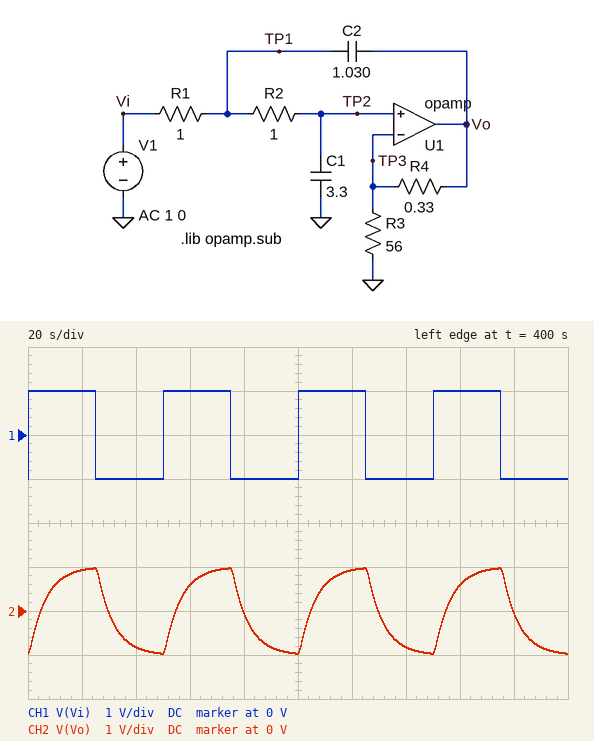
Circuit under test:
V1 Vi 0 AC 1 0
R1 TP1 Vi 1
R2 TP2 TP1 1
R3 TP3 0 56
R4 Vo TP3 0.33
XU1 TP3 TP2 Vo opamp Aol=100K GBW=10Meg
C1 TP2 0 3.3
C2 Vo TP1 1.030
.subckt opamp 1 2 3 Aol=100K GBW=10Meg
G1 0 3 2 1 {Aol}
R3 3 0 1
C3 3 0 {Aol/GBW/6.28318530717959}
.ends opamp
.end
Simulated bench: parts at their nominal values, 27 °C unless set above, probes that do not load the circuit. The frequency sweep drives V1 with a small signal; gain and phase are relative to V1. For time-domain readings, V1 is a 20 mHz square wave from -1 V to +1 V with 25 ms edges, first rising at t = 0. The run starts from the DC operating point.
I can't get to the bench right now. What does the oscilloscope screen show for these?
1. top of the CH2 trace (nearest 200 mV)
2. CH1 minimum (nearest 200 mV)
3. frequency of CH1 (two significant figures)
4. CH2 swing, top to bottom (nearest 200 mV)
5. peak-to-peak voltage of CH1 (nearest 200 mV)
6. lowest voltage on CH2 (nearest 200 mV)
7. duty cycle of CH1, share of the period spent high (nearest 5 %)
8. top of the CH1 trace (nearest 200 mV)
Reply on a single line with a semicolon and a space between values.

1.0 V; -1.0 V; 20 mHz; 2.0 V; 2.0 V; -1.0 V; 50 %; 1.0 V
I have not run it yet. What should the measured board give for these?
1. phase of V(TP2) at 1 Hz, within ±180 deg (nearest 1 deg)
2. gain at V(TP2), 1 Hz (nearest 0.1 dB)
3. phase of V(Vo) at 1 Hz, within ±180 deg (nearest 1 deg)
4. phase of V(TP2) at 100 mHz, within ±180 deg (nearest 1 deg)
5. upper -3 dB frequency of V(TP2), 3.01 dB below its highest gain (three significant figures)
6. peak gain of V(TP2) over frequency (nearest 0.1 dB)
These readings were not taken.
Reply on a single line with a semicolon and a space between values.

-163 deg; -42.9 dB; -163 deg; -95 deg; 26.2 mHz; 0 dB
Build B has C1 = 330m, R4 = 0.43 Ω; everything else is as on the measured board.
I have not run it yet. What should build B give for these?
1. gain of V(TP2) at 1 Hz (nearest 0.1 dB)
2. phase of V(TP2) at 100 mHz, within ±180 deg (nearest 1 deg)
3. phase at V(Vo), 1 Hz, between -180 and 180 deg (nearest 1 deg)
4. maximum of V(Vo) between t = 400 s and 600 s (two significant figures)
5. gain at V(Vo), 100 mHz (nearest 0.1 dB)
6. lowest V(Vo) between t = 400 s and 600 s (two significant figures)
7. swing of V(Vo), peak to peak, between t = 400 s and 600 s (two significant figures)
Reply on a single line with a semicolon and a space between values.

-22.3 dB; -25 deg; -162 deg; 1.3 V; 0.4 dB; -1.3 V; 2.5 V
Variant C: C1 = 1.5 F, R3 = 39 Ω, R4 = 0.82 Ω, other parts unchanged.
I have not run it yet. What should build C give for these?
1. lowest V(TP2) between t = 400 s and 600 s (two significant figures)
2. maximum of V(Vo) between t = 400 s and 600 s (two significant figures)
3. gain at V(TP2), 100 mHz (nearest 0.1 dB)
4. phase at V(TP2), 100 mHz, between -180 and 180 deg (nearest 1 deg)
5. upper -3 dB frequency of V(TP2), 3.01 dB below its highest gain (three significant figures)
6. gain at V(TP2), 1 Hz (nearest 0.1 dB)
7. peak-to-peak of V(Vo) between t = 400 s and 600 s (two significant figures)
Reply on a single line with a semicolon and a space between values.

-1.0 V; 1.0 V; -5.6 dB; -78 deg; 64.1 mHz; -36.0 dB; 2.0 V
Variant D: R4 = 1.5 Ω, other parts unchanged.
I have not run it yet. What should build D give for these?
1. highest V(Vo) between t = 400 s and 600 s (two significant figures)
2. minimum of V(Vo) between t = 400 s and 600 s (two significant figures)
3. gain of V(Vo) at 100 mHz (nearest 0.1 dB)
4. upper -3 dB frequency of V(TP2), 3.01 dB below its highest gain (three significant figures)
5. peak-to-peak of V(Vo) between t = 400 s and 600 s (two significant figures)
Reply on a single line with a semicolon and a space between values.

990 mV; -990 mV; -12.1 dB; 26.3 mHz; 2.0 V
